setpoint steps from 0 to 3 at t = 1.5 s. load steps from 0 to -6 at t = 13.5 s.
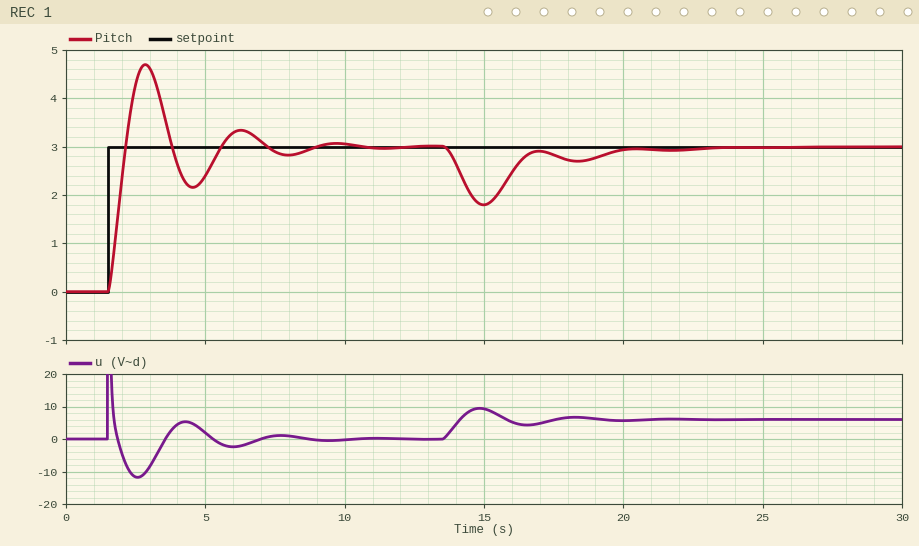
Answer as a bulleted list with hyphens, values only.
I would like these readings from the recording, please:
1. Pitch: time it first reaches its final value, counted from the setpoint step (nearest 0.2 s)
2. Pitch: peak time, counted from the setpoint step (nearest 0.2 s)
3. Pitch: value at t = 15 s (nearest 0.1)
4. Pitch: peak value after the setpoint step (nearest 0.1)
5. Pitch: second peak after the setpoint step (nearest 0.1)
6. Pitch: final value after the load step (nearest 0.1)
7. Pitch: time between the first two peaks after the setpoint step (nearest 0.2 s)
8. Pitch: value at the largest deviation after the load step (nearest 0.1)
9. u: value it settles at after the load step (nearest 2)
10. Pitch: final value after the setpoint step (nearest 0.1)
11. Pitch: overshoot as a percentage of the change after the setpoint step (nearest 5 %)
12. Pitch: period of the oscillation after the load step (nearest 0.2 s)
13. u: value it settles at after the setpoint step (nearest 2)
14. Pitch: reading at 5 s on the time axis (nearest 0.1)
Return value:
- 0.6 s
- 1.4 s
- 1.8
- 4.7
- 3.3
- 3.0
- 3.4 s
- 1.8
- 6
- 3.0
- 55 %
- 3.4 s
- 0
- 2.4
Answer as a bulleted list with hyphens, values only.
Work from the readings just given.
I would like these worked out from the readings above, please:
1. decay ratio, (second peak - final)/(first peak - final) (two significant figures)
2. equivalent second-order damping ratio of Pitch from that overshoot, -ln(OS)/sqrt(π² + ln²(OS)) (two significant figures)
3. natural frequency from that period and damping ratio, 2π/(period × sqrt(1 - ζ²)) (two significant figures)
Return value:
- 0.18
- 0.19
- 1.9 rad/s
